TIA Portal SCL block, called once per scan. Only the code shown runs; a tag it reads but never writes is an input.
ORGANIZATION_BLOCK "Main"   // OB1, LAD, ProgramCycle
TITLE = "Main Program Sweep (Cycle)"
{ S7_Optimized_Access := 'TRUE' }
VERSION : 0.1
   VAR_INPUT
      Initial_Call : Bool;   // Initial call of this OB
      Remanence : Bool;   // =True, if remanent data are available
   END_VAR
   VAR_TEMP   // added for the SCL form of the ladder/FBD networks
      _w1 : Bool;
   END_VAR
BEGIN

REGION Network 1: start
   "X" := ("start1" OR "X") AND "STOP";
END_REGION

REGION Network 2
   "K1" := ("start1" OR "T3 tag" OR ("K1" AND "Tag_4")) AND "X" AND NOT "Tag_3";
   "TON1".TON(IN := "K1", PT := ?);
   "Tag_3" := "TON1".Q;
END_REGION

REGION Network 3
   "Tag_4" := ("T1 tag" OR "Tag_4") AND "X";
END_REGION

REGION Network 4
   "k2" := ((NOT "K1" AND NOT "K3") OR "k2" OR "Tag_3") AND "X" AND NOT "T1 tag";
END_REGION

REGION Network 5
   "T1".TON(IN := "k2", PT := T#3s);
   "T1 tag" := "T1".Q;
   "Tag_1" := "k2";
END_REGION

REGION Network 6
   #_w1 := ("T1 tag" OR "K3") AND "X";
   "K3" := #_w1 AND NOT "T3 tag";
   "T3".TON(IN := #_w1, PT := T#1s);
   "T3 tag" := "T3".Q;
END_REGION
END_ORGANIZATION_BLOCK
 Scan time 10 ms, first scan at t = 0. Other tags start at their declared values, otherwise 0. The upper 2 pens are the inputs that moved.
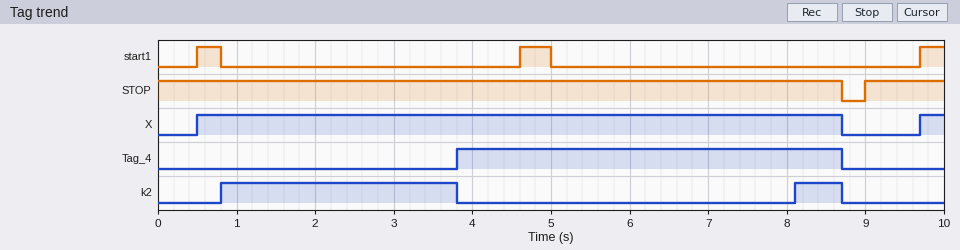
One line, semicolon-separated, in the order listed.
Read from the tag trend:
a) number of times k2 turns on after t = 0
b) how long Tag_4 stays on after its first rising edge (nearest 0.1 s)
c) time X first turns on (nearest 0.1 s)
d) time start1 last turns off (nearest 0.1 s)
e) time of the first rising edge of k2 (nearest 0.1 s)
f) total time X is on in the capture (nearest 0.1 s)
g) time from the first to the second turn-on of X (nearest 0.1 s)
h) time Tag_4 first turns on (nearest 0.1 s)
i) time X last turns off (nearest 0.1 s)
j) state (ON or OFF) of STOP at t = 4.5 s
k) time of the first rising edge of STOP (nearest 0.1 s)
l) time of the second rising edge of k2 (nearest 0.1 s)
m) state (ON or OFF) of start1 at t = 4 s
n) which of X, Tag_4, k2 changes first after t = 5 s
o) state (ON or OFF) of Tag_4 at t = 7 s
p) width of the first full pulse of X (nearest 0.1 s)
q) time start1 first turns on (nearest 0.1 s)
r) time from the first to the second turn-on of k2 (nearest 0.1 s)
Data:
2; 4.9 s; 0.5 s; 5.0 s; 0.8 s; 8.5 s; 9.2 s; 3.8 s; 8.7 s; ON; 9.0 s; 8.1 s; OFF; k2; ON; 8.2 s; 0.5 s; 7.3 s
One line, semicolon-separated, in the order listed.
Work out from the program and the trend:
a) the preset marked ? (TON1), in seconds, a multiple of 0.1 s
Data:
3.5 s
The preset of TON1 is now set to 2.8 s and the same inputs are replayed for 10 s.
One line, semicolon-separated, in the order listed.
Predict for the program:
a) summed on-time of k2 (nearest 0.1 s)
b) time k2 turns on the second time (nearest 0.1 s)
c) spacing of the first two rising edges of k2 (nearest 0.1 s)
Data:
4.3 s; 7.4 s; 6.6 s
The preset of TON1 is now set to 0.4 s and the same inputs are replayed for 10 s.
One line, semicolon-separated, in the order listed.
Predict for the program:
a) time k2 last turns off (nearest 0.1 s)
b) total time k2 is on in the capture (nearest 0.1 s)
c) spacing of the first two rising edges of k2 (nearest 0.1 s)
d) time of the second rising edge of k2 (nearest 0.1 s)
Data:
8.0 s; 6.0 s; 4.2 s; 5.0 s
